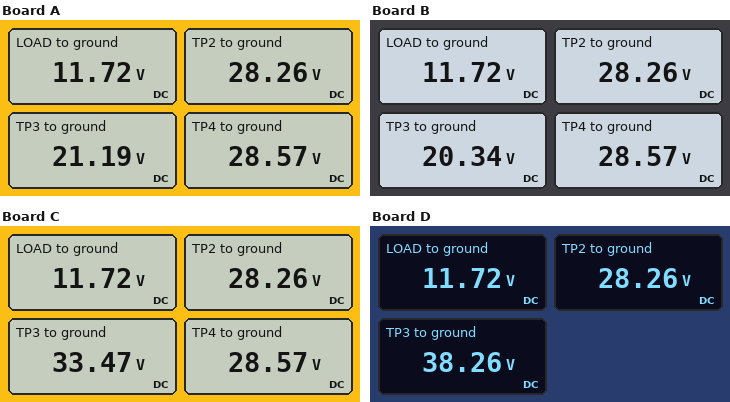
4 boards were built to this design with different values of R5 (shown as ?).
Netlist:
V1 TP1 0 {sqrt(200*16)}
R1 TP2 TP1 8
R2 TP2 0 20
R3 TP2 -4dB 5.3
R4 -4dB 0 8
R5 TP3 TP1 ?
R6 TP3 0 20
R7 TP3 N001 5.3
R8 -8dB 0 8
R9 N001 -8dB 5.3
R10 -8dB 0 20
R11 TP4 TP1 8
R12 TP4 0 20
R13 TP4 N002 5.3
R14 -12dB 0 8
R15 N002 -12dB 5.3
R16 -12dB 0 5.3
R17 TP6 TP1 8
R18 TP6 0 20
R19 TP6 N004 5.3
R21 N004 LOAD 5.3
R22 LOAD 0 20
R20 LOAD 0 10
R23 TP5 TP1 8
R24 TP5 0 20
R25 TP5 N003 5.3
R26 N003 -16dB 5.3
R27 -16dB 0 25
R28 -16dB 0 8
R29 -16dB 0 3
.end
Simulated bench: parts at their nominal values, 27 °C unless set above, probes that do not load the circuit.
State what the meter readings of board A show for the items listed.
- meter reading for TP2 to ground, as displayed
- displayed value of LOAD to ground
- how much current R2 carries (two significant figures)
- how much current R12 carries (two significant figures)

28.26 V
11.72 V
1.4 A
1.4 A
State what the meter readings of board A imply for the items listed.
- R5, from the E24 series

15 Ω
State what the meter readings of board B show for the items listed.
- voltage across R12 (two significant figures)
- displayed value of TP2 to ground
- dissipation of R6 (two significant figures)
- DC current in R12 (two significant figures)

29 V
28.26 V
21 W
1.4 A
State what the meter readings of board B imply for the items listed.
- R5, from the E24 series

16 Ω
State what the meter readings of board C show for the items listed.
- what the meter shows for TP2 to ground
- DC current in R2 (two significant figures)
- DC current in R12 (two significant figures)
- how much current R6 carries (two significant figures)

28.26 V
1.4 A
1.4 A
1.7 A
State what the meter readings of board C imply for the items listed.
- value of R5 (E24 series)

6.2 Ω
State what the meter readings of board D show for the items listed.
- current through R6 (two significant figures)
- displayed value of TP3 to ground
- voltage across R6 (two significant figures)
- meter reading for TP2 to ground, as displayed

1.9 A
38.26 V
38 V
28.26 V
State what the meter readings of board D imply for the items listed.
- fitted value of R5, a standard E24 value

4.3 Ω
